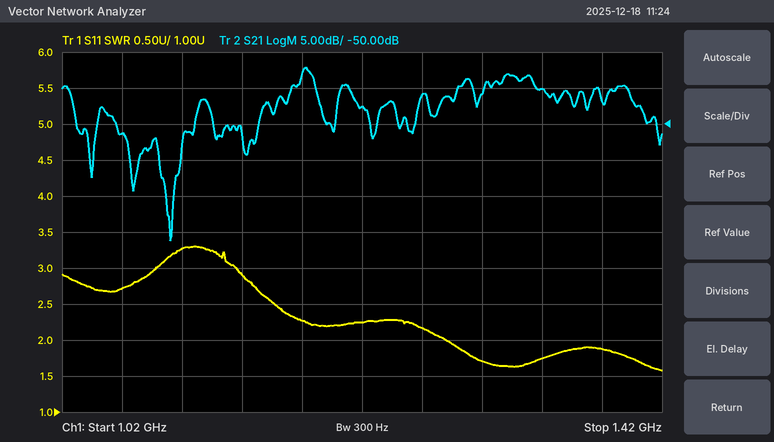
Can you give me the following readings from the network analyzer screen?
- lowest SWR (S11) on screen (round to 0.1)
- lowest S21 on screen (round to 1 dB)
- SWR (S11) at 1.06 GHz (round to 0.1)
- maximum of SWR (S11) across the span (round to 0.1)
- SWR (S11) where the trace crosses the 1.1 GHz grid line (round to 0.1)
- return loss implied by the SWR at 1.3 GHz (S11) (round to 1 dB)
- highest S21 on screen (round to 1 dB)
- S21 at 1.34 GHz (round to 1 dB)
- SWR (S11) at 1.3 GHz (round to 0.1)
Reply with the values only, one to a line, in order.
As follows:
1.6
-66 dB
2.7
3.3
3.3
12 dB
-42 dB
-45 dB
1.7
